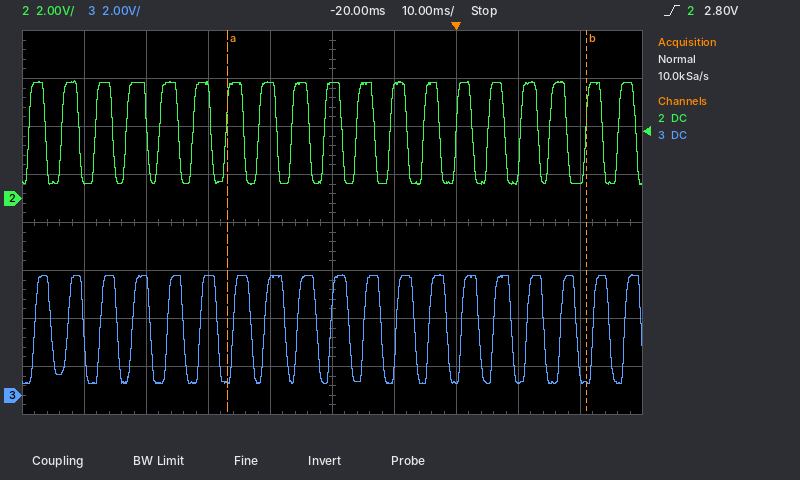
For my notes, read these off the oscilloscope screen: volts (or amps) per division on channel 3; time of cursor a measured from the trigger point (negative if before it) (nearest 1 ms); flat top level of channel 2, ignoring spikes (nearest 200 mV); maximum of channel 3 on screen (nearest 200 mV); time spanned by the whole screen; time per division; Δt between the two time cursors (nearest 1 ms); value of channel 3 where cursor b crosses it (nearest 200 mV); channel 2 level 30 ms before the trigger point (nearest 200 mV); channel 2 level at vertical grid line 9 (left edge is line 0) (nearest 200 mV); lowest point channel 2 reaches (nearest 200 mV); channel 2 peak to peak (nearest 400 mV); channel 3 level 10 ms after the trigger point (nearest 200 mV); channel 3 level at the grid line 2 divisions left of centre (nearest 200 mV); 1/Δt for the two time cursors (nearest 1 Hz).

2 V
-37 ms
4.8 V
5.0 V
100 ms
10 ms
58 ms
600 mV
4.8 V
800 mV
600 mV
4.4 V
600 mV
5.0 V
17 Hz
